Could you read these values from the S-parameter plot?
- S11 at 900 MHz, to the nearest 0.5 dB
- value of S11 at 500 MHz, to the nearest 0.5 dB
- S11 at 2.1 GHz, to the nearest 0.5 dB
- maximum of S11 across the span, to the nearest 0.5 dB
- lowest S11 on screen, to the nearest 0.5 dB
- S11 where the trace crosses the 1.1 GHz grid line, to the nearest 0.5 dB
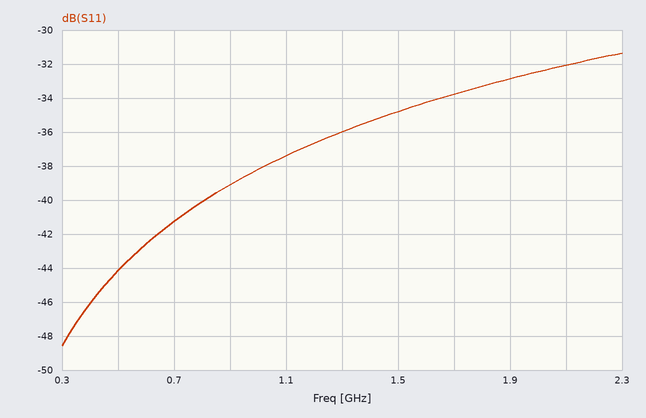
-39.0 dB
-44.0 dB
-32.0 dB
-31.5 dB
-48.5 dB
-37.5 dB
